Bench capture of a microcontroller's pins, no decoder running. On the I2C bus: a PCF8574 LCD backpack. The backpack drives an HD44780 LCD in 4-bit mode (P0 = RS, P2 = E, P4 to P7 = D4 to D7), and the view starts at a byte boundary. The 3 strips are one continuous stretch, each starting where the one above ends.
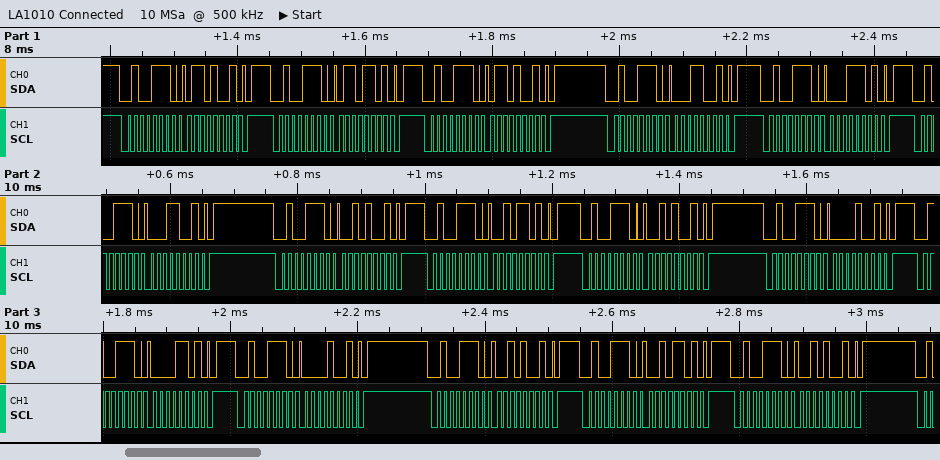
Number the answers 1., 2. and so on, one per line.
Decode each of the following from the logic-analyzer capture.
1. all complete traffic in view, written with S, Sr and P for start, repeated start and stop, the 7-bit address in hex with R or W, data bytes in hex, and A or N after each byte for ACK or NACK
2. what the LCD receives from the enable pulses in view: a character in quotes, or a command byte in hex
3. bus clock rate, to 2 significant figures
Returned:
1. S 27W A 69 A P S 27W A 6D A P S 27W A 69 A P S 27W A 19 A P S 27W A 1D A P S 27W A 19 A P S 27W A 29 A P S 27W A 2D A P S 27W A 29 A P S 27W A 09 A P S 27W A 0D A P S 27W A 09 A P S 27W A 29 A P S 27W A 2D A P S 27W A 29 A P
2. 'a' ' '
3. 100 kHz
